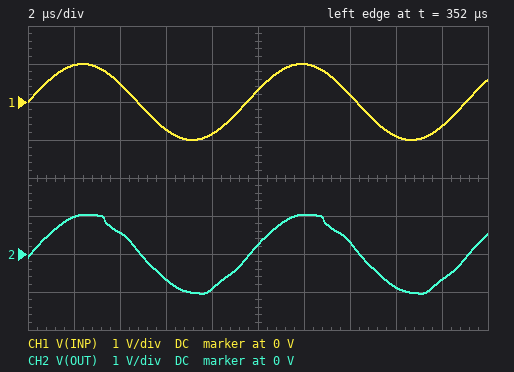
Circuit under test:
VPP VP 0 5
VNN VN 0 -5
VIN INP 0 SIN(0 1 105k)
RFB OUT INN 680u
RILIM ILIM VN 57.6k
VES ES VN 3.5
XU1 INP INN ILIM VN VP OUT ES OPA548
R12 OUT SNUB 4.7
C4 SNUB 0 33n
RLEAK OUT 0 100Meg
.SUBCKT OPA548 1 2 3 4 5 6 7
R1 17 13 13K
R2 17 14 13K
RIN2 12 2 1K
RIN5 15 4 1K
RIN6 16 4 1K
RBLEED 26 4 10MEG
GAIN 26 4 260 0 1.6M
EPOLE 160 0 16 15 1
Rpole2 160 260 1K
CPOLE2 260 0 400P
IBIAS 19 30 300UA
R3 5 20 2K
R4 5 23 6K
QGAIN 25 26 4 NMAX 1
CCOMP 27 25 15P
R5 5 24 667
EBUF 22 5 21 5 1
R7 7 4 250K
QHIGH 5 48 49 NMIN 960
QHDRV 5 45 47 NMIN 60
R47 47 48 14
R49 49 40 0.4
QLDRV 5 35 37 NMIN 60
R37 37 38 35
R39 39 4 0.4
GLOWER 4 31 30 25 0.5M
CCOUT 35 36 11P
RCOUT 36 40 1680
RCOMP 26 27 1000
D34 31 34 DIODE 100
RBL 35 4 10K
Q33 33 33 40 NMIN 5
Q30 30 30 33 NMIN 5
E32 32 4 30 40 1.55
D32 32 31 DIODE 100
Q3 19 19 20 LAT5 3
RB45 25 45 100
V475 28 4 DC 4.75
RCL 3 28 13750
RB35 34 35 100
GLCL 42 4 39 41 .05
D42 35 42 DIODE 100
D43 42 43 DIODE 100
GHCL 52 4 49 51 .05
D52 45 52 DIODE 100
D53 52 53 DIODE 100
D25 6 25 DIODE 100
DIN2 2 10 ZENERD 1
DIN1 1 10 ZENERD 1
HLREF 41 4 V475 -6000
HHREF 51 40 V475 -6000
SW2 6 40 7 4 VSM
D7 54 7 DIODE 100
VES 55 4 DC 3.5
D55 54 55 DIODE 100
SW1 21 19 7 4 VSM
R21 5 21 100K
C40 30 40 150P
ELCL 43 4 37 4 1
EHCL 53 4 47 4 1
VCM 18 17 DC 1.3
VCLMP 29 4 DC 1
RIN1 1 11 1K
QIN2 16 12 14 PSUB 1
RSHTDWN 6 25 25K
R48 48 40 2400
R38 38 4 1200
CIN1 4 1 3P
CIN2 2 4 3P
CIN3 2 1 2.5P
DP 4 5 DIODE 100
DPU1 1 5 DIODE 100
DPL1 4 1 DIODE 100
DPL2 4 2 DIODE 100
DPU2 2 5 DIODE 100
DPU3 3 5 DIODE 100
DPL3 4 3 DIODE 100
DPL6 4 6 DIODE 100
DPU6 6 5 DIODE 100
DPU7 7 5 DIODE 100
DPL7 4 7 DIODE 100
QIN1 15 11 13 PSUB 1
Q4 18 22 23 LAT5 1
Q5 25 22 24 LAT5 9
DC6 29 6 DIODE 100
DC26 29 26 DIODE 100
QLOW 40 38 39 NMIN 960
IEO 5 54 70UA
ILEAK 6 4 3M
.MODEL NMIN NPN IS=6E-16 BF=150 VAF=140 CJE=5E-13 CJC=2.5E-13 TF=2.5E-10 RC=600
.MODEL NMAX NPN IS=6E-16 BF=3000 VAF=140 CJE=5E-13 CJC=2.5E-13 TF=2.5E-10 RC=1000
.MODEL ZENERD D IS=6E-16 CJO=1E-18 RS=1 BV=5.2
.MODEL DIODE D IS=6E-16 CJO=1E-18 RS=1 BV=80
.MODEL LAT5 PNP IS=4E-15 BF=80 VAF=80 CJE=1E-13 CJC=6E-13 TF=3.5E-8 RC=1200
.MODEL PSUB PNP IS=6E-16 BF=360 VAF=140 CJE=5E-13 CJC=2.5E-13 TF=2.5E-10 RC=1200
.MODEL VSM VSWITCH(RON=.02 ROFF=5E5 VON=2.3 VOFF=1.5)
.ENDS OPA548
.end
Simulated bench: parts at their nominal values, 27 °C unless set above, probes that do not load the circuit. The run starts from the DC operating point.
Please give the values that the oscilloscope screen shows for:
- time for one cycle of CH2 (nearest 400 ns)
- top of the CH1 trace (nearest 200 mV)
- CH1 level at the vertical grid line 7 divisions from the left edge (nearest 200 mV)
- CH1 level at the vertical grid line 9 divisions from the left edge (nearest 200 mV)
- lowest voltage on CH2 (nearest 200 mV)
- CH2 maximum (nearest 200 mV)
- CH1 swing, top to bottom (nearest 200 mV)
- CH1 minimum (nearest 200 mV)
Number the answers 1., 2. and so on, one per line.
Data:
1. 9.6 µs
2. 1.0 V
3. 200 mV
4. -600 mV
5. -1.0 V
6. 1.0 V
7. 2.0 V
8. -1.0 V
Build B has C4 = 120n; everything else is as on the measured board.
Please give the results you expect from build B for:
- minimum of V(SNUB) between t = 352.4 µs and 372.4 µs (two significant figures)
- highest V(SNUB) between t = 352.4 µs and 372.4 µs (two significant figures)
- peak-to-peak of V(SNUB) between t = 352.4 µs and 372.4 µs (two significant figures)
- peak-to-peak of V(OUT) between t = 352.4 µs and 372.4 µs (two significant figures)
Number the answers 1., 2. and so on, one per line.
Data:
1. -970 mV
2. 980 mV
3. 1.9 V
4. 2.1 V
